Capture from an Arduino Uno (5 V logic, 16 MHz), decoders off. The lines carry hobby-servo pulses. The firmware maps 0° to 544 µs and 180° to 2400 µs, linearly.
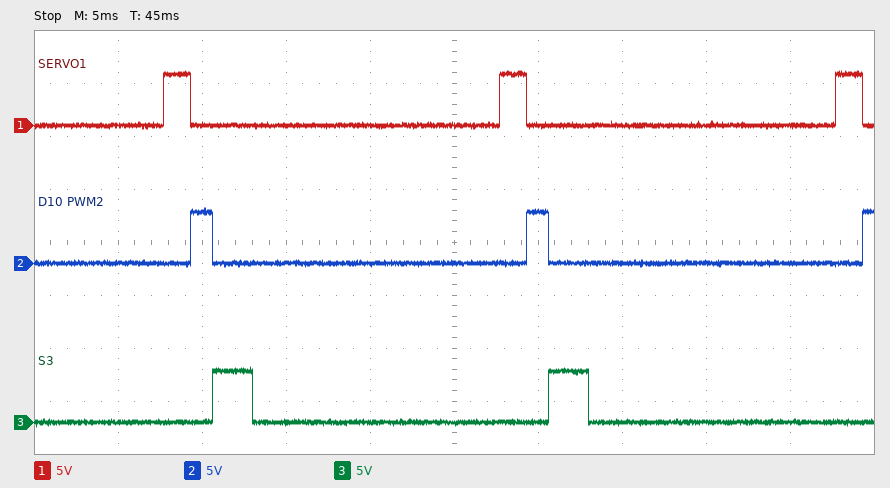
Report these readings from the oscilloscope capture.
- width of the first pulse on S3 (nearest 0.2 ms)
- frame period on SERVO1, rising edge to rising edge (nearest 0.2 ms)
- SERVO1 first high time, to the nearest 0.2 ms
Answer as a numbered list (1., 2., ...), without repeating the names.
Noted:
1. 2.4 ms
2. 20.0 ms
3. 1.6 ms
